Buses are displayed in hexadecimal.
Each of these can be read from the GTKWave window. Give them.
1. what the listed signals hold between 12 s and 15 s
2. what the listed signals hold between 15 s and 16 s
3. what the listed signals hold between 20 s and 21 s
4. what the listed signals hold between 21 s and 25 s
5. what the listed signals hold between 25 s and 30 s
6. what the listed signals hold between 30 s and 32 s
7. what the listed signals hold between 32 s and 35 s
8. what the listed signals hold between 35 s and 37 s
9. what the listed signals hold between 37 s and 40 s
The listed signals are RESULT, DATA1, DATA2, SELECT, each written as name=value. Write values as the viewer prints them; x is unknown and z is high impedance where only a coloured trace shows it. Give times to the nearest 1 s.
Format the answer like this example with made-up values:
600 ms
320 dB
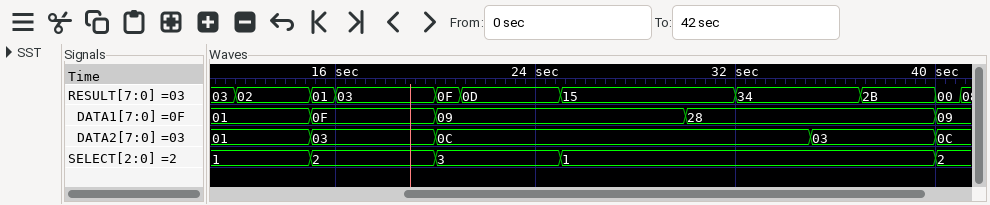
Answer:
RESULT=02, DATA1=01, DATA2=01, SELECT=1
RESULT=01, DATA1=0F, DATA2=03, SELECT=2
RESULT=0F, DATA1=09, DATA2=0C, SELECT=3
RESULT=0D, DATA1=09, DATA2=0C, SELECT=3
RESULT=15, DATA1=09, DATA2=0C, SELECT=1
RESULT=15, DATA1=28, DATA2=0C, SELECT=1
RESULT=34, DATA1=28, DATA2=0C, SELECT=1
RESULT=34, DATA1=28, DATA2=03, SELECT=1
RESULT=2B, DATA1=28, DATA2=03, SELECT=1
